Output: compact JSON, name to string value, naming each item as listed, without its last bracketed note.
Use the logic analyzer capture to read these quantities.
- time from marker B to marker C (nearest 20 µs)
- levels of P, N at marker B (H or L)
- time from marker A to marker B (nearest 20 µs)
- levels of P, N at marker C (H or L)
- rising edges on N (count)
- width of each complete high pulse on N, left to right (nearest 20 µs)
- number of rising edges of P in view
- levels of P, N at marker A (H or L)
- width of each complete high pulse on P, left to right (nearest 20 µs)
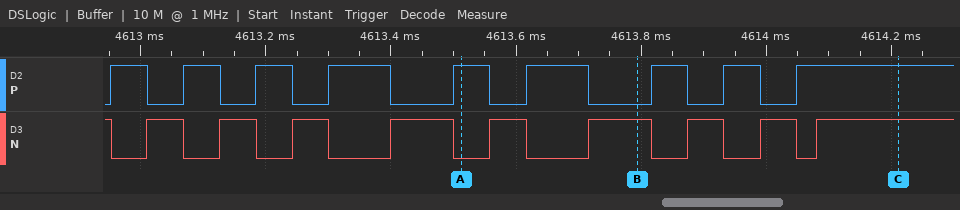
{"time from marker B to marker C": "420 µs", "levels of P, N at marker B": "P=L, N=H", "time from marker A to marker B": "280 µs", "levels of P, N at marker C": "P=H, N=H", "rising edges on N": "9", "width of each complete high pulse on N, left to right": "60 µs, 60 µs, 60 µs, 100 µs, 60 µs, 100 µs, 60 µs, 60 µs", "number of rising edges of P in view": "9", "levels of P, N at marker A": "P=H, N=L", "width of each complete high pulse on P, left to right": "60 µs, 60 µs, 60 µs, 100 µs, 60 µs, 100 µs, 60 µs, 60 µs"}
